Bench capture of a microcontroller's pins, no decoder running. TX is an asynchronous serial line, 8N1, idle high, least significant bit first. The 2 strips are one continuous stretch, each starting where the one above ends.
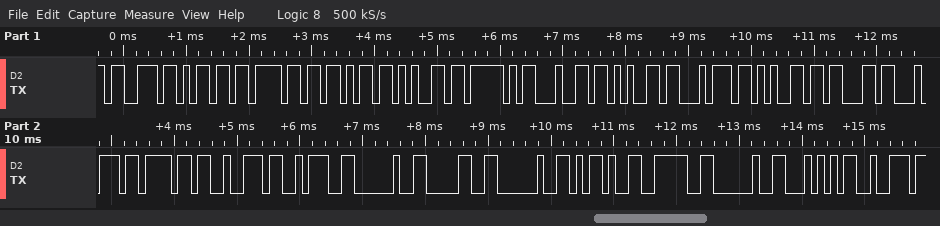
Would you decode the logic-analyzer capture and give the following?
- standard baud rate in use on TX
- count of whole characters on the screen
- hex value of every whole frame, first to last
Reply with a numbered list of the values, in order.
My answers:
1. 9600 baud
2. 23
3. 73 6D 6F 6B 65 5F 64 65 74 65 63 74 6F 72 3A 20 30 20 2D 3E 20 54 72
